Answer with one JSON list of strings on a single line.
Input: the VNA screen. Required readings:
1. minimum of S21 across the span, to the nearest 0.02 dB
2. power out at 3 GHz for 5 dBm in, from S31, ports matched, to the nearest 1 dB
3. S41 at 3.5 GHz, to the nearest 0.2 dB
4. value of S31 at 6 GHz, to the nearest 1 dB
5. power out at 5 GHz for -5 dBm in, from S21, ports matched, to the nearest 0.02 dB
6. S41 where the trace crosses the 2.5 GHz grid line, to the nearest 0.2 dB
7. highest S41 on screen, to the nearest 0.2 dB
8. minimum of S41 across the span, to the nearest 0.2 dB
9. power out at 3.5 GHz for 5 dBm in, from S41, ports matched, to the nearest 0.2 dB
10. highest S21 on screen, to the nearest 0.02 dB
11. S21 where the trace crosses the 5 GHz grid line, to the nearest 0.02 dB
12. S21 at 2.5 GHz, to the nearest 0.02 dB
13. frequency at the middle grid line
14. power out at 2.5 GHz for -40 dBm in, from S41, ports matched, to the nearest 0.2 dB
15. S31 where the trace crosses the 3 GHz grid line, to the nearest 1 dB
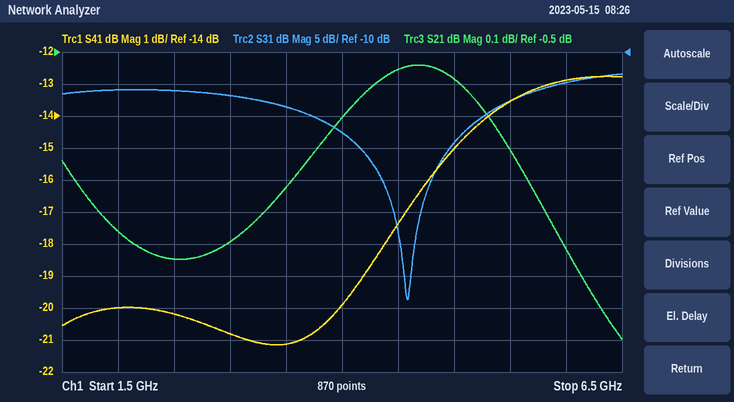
["-1.40 dB", "-12 dBm", "-21.2 dB", "-15 dB", "-5.58 dBm", "-20.2 dB", "-12.8 dB", "-21.2 dB", "-16.2 dBm", "-0.54 dB", "-0.58 dB", "-1.14 dB", "4 GHz", "-60.2 dBm", "-17 dB"]
